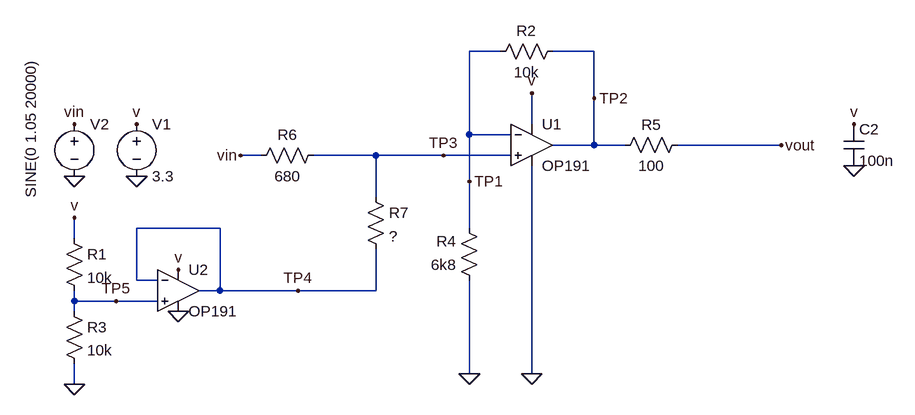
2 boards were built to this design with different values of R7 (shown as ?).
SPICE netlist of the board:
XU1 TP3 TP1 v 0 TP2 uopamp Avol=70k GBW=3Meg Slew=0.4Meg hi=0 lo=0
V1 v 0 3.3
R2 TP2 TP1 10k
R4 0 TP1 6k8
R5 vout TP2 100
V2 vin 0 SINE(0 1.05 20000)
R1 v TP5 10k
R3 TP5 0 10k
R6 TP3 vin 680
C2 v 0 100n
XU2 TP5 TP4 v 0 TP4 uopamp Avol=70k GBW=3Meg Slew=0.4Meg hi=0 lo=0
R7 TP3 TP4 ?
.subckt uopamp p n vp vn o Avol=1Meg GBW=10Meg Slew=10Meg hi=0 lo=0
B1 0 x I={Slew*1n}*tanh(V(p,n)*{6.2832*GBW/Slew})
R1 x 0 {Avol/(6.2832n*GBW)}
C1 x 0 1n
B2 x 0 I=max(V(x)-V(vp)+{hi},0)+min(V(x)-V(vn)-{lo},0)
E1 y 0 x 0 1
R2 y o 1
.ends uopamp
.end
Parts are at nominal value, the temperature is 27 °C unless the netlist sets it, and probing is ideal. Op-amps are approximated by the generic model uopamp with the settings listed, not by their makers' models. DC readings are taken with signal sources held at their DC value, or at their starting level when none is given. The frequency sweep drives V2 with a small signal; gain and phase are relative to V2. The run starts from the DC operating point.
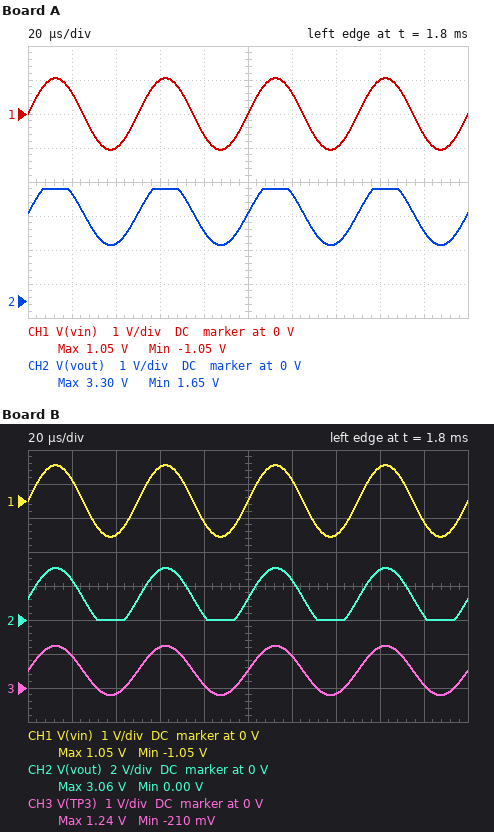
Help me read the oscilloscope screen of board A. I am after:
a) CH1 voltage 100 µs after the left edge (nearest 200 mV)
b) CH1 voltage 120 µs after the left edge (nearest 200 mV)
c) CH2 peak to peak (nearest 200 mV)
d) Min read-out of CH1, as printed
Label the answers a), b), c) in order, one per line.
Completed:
a) 0 V
b) 600 mV
c) 1.6 V
d) -1.05 V
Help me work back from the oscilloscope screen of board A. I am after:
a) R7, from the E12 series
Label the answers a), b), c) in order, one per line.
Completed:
a) 390 Ω
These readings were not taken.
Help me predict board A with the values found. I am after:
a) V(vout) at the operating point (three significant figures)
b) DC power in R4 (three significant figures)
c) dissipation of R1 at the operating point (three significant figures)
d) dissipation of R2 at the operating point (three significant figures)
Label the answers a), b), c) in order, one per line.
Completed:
a) 2.59 V
b) 162 µW
c) 272 µW
d) 238 µW
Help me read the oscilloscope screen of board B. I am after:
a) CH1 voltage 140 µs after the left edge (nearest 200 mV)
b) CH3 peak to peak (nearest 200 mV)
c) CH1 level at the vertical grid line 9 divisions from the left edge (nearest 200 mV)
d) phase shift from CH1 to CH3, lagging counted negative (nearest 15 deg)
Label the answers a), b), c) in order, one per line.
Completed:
a) -1.0 V
b) 1.4 V
c) -600 mV
d) 0 deg
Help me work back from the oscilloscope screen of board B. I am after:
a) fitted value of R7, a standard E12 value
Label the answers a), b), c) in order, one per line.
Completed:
a) 1.5 kΩ
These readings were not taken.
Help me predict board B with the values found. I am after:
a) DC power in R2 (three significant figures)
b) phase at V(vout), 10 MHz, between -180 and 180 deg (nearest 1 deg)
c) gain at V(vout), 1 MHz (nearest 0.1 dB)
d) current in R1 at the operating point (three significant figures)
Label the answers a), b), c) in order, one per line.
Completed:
a) 57.3 µW
b) -83 deg
c) 2.4 dB
d) 165 µA
